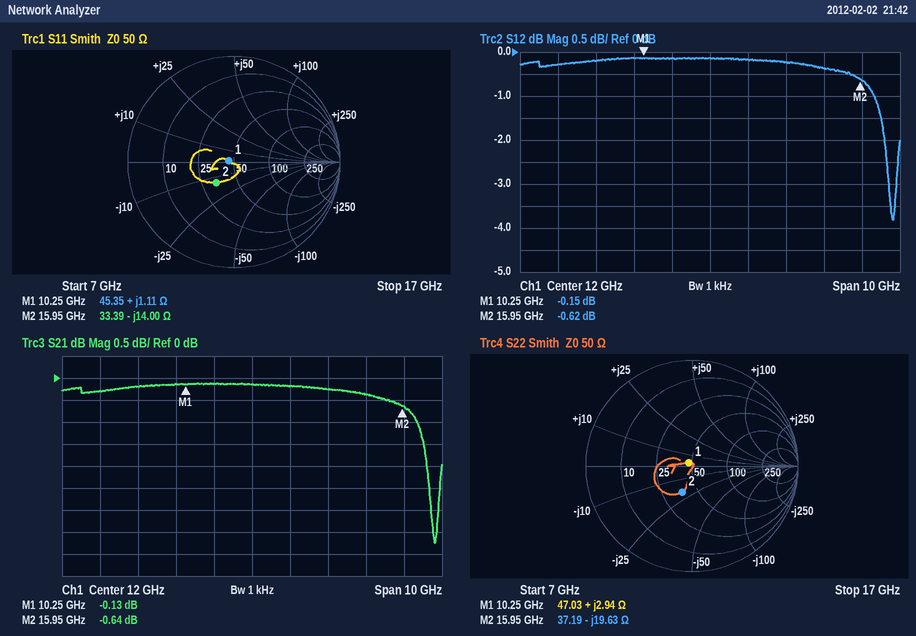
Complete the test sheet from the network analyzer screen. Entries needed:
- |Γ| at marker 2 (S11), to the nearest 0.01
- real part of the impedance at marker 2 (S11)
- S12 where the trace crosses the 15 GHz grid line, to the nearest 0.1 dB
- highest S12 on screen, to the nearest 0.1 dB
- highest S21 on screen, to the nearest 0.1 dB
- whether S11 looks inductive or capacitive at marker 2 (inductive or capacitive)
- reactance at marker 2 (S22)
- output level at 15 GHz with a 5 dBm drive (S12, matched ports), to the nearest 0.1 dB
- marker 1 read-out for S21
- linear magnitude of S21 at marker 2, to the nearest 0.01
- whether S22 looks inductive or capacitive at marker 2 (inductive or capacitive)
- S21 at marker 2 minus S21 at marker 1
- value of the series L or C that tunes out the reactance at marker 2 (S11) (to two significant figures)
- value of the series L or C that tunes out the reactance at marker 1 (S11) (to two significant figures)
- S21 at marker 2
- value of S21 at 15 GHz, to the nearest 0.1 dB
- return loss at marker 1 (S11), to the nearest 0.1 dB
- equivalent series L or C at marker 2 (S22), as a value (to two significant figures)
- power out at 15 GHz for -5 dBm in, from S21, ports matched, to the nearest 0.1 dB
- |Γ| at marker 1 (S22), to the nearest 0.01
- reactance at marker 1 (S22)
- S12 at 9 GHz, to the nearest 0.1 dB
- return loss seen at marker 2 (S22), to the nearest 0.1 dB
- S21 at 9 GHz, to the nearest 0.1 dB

0.26
33.39 Ω
-0.4 dB
-0.1 dB
-0.1 dB
capacitive
-19.63 Ω
4.6 dBm
-0.13 dB
0.93
capacitive
-0.51 dB
140 pH
14 pF
-0.64 dB
-0.4 dB
26.0 dB
510 fF
-5.4 dBm
0.04
+2.94 Ω
-0.2 dB
11.6 dB
-0.2 dB
